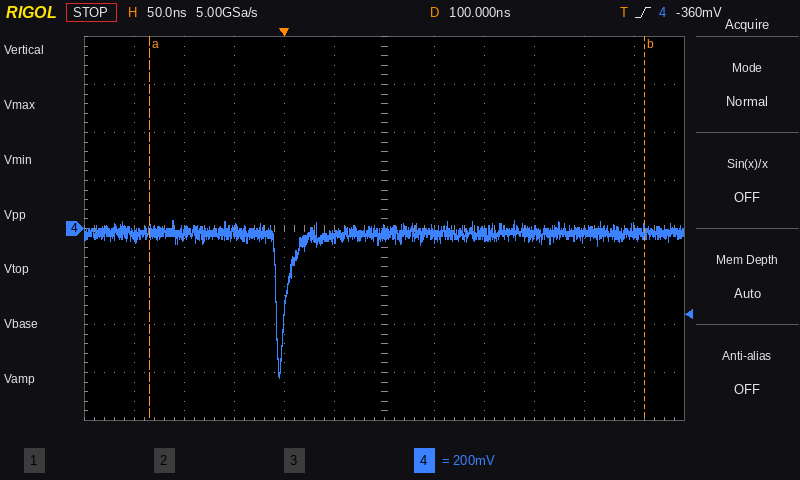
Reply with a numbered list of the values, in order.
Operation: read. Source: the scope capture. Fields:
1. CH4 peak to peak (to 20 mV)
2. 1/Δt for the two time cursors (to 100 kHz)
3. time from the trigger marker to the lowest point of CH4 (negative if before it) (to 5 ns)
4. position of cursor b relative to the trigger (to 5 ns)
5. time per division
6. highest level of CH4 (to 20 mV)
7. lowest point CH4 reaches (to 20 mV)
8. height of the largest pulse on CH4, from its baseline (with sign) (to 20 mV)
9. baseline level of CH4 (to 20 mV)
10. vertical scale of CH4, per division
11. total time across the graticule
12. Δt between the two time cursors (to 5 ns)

1. 660 mV
2. 2.0 MHz
3. -5 ns
4. +360 ns
5. 50 ns
6. 40 mV
7. -620 mV
8. -600 mV
9. -20 mV
10. 200 mV
11. 600 ns
12. 495 ns
